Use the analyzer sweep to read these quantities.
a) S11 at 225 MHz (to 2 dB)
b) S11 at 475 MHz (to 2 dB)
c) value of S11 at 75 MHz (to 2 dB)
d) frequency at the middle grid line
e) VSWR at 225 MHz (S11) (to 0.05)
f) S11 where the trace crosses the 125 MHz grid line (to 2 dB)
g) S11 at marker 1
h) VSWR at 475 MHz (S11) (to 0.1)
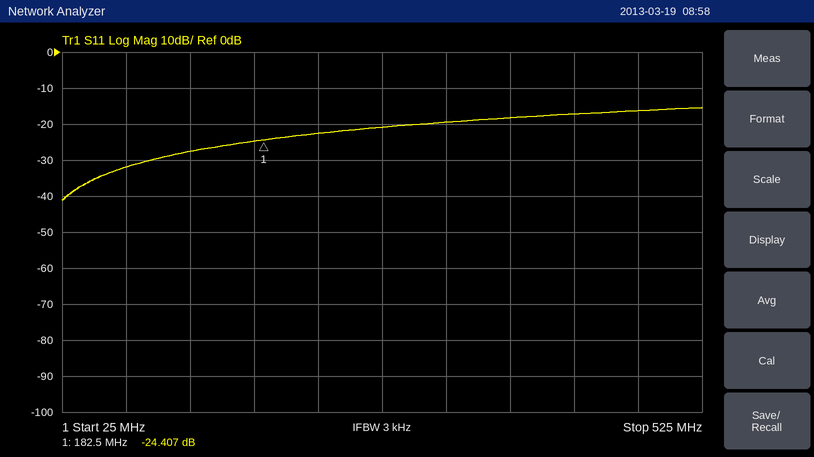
-22 dB
-16 dB
-32 dB
275 MHz
1.15
-28 dB
-24.407 dB
1.4
